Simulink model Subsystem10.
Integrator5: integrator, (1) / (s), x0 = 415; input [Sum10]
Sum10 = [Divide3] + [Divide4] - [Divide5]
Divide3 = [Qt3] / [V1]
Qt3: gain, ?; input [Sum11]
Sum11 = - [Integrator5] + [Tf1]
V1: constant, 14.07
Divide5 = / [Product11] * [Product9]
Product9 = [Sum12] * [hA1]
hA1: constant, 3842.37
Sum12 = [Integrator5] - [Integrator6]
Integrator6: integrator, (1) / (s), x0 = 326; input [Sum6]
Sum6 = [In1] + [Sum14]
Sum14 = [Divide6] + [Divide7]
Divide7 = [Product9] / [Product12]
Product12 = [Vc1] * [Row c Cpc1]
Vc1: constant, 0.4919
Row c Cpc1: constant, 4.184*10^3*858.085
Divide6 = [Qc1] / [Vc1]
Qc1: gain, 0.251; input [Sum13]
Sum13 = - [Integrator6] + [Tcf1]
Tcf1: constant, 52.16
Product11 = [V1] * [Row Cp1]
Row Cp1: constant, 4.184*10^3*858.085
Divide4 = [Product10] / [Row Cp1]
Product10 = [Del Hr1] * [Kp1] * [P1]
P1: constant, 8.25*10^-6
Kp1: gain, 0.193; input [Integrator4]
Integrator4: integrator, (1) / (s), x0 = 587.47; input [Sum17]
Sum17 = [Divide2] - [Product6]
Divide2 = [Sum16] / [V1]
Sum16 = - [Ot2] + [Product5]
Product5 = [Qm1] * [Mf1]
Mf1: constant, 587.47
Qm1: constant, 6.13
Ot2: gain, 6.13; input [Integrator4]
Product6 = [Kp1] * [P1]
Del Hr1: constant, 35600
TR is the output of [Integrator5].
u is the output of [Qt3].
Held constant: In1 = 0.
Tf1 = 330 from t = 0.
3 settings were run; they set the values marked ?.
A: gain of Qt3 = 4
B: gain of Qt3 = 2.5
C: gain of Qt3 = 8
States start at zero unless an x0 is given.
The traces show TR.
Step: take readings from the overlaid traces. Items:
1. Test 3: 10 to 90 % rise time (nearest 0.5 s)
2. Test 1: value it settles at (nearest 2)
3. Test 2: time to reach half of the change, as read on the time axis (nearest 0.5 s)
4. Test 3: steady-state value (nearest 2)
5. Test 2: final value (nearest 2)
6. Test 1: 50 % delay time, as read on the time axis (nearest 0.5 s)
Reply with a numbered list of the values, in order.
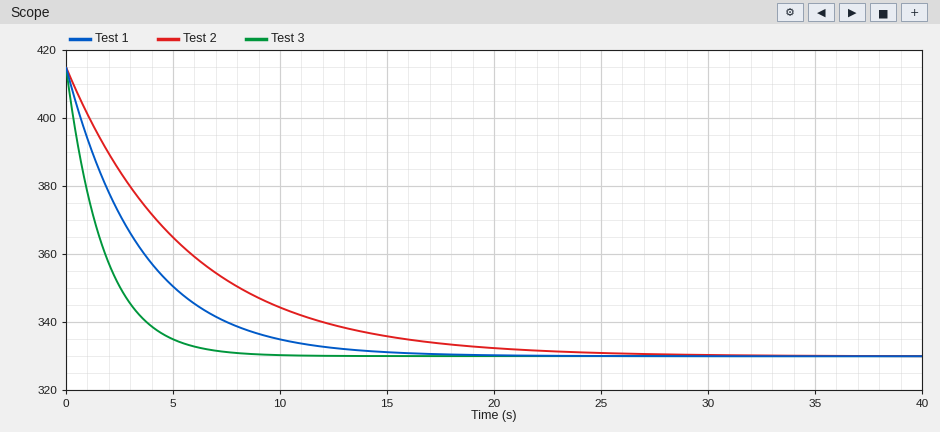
1. 4.0 s
2. 330
3. 4.0 s
4. 330
5. 330
6. 2.5 s
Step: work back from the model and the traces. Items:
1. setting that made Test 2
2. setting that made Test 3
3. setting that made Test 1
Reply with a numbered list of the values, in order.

1. B
2. C
3. A
